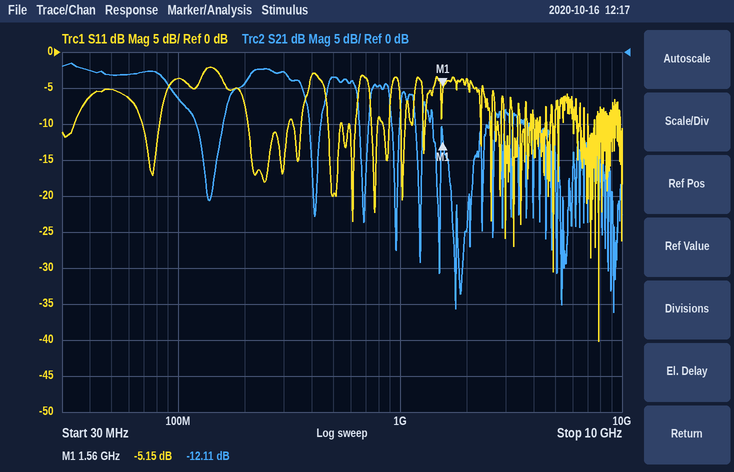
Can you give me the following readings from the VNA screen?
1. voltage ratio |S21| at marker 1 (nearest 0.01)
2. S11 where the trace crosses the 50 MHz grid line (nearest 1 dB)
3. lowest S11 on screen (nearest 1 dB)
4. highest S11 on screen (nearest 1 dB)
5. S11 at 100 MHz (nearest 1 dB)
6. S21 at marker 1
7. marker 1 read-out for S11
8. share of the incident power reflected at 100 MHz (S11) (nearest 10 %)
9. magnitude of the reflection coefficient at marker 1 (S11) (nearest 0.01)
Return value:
0.25
-5 dB
-40 dB
-2 dB
-4 dB
-12.11 dB
-5.15 dB
40 %
0.55
